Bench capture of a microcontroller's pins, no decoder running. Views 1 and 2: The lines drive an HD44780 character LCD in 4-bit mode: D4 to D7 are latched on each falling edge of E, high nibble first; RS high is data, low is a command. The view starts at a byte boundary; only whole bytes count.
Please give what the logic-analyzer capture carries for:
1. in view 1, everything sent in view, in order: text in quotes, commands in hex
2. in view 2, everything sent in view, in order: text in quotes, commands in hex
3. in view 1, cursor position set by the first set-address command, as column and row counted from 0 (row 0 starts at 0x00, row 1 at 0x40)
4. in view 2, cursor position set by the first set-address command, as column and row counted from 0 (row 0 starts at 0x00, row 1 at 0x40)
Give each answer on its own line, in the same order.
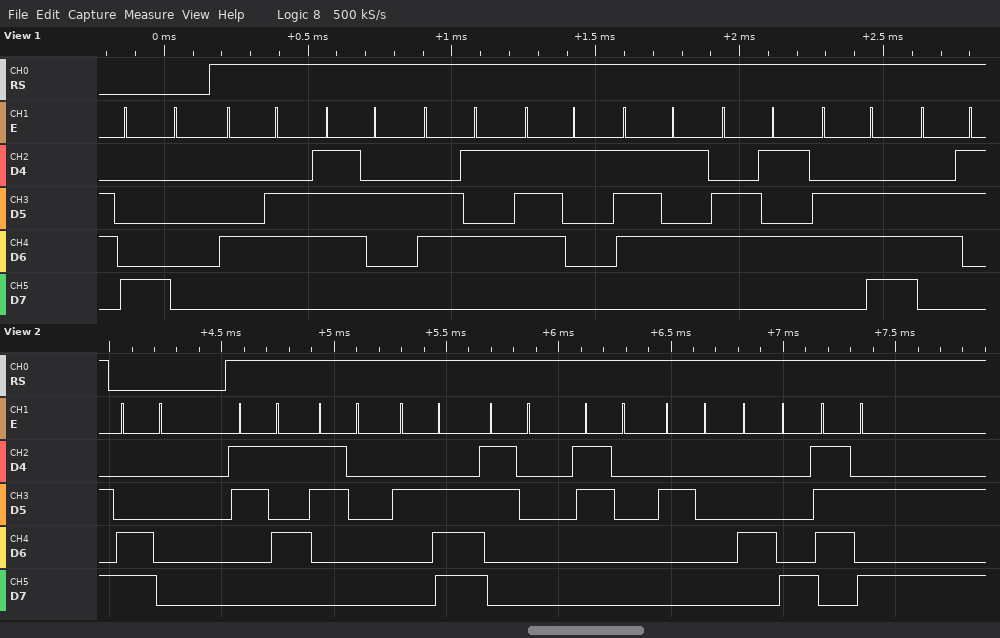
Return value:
0x80 "Frequenc"
0xC0 "50.00 Hz"
column 0, row 0
column 0, row 1
